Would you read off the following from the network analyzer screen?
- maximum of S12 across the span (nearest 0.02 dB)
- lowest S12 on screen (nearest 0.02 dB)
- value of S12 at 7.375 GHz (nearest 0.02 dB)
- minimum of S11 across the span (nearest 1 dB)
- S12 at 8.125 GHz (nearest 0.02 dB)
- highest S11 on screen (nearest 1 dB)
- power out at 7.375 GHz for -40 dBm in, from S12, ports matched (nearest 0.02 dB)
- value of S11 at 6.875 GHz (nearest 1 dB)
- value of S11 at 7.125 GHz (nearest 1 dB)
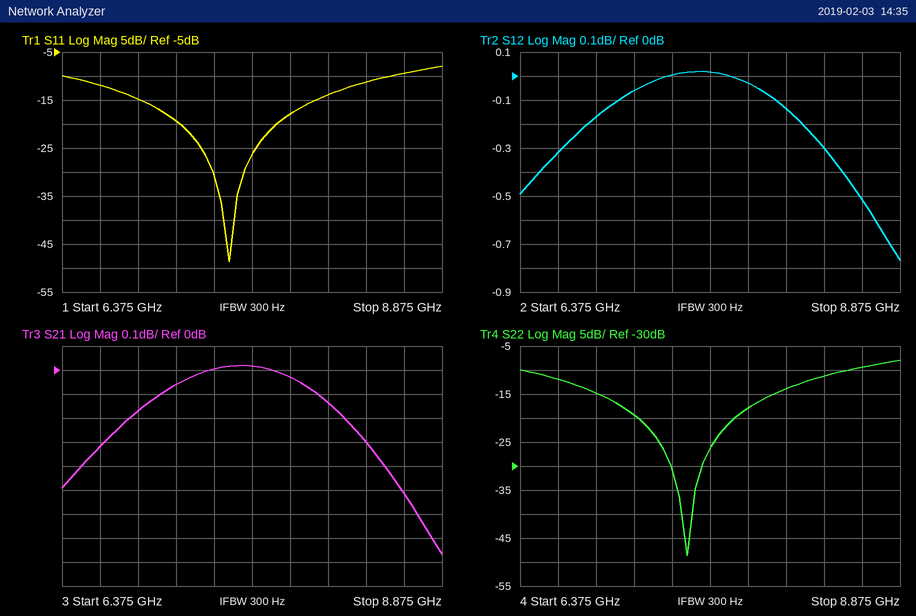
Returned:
0.02 dB
-0.76 dB
0.00 dB
-49 dB
-0.14 dB
-8 dB
-40.00 dBm
-15 dB
-19 dB
